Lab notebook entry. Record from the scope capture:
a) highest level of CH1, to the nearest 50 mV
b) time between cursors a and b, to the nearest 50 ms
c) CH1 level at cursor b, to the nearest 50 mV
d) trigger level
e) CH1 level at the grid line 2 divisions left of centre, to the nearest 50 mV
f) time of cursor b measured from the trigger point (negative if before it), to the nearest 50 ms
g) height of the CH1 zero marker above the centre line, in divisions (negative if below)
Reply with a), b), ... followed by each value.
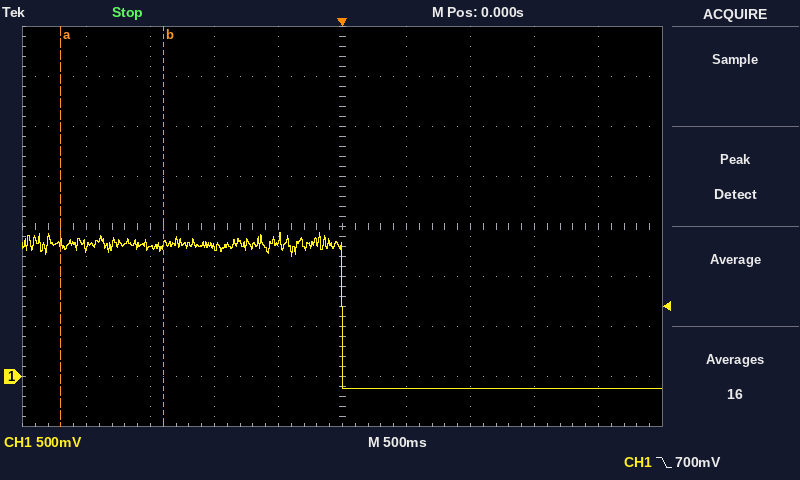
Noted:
a) 1.45 V
b) 800 ms
c) 1.30 V
d) 700 mV
e) 1.30 V
f) -1.40 s
g) -3.0 div
